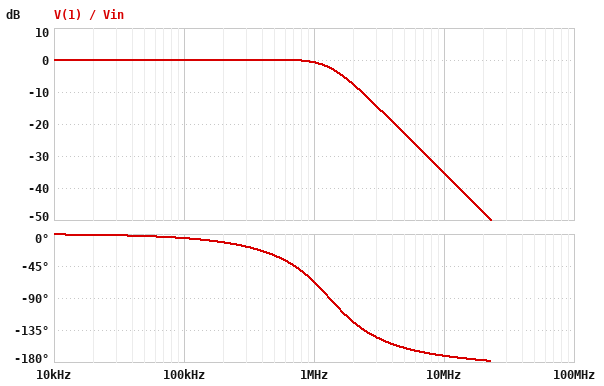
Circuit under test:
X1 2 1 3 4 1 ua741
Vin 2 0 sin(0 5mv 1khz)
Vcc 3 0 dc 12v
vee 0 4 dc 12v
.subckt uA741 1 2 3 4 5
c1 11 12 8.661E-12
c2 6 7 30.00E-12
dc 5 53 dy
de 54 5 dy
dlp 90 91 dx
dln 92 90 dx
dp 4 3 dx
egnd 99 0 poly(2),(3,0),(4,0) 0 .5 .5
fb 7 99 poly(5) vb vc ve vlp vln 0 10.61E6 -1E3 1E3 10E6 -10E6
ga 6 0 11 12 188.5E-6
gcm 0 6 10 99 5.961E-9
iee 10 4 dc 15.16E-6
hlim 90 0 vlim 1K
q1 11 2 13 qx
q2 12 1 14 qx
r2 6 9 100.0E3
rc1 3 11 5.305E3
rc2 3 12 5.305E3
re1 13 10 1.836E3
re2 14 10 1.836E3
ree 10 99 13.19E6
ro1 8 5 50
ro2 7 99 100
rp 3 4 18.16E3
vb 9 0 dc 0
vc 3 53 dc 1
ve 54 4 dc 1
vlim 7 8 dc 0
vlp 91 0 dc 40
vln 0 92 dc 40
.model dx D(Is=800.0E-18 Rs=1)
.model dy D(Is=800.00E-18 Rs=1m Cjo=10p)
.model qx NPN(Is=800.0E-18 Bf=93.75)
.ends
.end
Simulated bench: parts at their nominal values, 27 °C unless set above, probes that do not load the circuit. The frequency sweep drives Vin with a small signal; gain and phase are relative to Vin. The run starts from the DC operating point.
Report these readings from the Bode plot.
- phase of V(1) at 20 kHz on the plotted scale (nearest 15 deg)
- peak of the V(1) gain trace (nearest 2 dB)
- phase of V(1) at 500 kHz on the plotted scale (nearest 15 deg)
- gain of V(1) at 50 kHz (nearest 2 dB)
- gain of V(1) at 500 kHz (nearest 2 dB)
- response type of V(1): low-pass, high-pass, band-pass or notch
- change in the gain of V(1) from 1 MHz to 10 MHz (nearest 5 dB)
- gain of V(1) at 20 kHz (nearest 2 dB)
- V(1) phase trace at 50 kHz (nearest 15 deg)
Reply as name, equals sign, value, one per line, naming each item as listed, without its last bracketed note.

phase of V(1) at 20 kHz on the plotted scale = 0 deg
peak of the V(1) gain trace = 0 dB
phase of V(1) at 500 kHz on the plotted scale = -30 deg
gain of V(1) at 50 kHz = 0 dB
gain of V(1) at 500 kHz = 0 dB
response type of V(1): low-pass, high-pass, band-pass or notch = low-pass
change in the gain of V(1) from 1 MHz to 10 MHz = -35 dB
gain of V(1) at 20 kHz = 0 dB
V(1) phase trace at 50 kHz = 0 deg
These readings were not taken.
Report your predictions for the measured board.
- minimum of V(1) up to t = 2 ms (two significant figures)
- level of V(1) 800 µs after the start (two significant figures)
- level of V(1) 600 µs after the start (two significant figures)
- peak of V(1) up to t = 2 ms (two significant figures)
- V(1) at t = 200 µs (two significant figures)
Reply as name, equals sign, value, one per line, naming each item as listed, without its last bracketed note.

minimum of V(1) up to t = 2 ms = -5.0 mV
level of V(1) 800 µs after the start = -4.7 mV
level of V(1) 600 µs after the start = -2.9 mV
peak of V(1) up to t = 2 ms = 5.0 mV
V(1) at t = 200 µs = 4.8 mV
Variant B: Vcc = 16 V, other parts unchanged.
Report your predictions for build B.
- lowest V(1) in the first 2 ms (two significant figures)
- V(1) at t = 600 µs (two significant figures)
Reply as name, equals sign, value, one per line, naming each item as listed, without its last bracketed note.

lowest V(1) in the first 2 ms = -4.9 mV
V(1) at t = 600 µs = -2.8 mV
